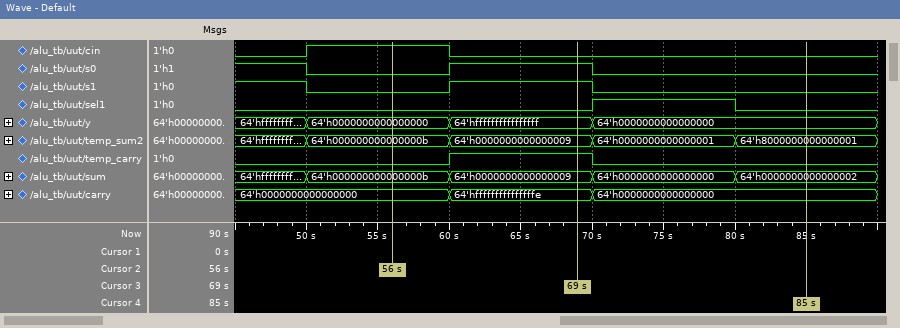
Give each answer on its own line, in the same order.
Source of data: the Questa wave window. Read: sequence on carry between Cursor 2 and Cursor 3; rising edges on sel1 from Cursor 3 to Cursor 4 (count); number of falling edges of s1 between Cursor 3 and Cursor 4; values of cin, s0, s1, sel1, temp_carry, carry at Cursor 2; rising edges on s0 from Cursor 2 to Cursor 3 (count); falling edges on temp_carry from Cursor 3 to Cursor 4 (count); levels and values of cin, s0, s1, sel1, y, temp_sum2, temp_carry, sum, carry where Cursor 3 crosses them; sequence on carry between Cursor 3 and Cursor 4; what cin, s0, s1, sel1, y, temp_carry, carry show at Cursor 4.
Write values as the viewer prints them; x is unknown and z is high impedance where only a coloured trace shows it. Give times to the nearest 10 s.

64'h0000000000000000, 64'hfffffffffffffffe
1
1
cin=1, s0=0, s1=0, sel1=0, temp_carry=0, carry=64'h0000000000000000
1
1
cin=0, s0=1, s1=1, sel1=0, y=64'hffffffffffffffff, temp_sum2=64'h0000000000000009, temp_carry=1, sum=64'h0000000000000009, carry=64'hfffffffffffffffe
64'hfffffffffffffffe, 64'h0000000000000000
cin=0, s0=0, s1=0, sel1=0, y=64'h0000000000000000, temp_carry=0, carry=64'h0000000000000000
